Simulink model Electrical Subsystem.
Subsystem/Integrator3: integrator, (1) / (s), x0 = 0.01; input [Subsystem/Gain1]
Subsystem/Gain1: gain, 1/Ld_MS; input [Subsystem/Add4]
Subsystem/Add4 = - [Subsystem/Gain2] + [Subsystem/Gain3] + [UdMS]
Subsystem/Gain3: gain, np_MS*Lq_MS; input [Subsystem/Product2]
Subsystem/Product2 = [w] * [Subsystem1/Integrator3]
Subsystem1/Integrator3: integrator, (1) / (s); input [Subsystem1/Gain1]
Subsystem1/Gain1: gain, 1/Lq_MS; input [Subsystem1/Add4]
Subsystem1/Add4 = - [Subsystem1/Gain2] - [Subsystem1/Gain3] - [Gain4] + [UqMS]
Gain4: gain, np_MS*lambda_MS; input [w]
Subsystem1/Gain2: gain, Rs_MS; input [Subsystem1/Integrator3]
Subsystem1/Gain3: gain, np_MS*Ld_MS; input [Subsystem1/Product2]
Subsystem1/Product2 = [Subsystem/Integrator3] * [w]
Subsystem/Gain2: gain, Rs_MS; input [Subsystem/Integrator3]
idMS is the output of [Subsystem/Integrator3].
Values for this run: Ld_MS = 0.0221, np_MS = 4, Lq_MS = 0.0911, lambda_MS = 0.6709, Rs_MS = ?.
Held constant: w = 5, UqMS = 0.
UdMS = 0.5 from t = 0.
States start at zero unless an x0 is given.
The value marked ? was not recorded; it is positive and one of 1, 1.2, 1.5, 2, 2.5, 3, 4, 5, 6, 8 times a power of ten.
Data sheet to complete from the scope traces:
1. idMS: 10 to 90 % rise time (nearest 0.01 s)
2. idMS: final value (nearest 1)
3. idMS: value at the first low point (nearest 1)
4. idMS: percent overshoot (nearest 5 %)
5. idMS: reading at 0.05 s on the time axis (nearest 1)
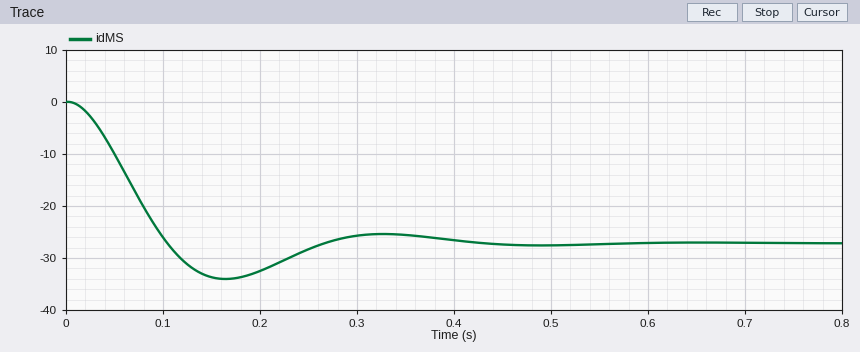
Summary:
0.07 s
-27
-34
25 %
-10
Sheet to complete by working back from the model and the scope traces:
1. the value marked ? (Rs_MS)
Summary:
0.3
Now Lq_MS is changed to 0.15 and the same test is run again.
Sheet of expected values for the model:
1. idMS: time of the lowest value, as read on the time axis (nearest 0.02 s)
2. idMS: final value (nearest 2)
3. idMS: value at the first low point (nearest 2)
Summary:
0.16 s
-28
-36
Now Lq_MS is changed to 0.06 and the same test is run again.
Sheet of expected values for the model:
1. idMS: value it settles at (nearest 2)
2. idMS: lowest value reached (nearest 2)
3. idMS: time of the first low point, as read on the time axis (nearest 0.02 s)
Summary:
-26
-32
0.16 s
